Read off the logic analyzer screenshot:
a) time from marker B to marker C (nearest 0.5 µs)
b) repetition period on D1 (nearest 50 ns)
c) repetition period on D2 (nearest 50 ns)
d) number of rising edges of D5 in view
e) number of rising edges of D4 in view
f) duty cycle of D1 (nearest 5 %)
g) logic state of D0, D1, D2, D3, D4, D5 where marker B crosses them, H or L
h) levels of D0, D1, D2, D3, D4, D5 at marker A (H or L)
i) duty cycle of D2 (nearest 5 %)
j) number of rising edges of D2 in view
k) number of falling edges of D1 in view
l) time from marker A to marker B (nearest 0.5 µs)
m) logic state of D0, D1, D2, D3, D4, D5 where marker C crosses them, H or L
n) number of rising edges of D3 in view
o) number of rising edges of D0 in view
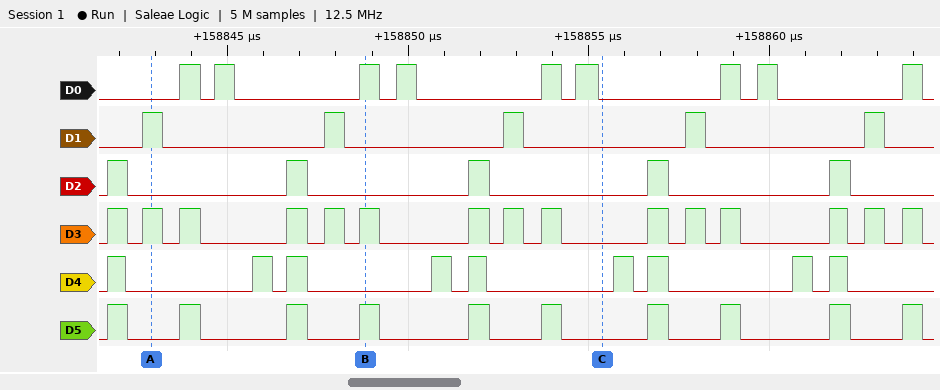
6.5 µs
5000 ns
5000 ns
10
9
10 %
D0=H, D1=L, D2=L, D3=H, D4=L, D5=H
D0=L, D1=H, D2=L, D3=H, D4=L, D5=L
10 %
5
5
6 µs
D0=L, D1=L, D2=L, D3=L, D4=L, D5=L
15
9
